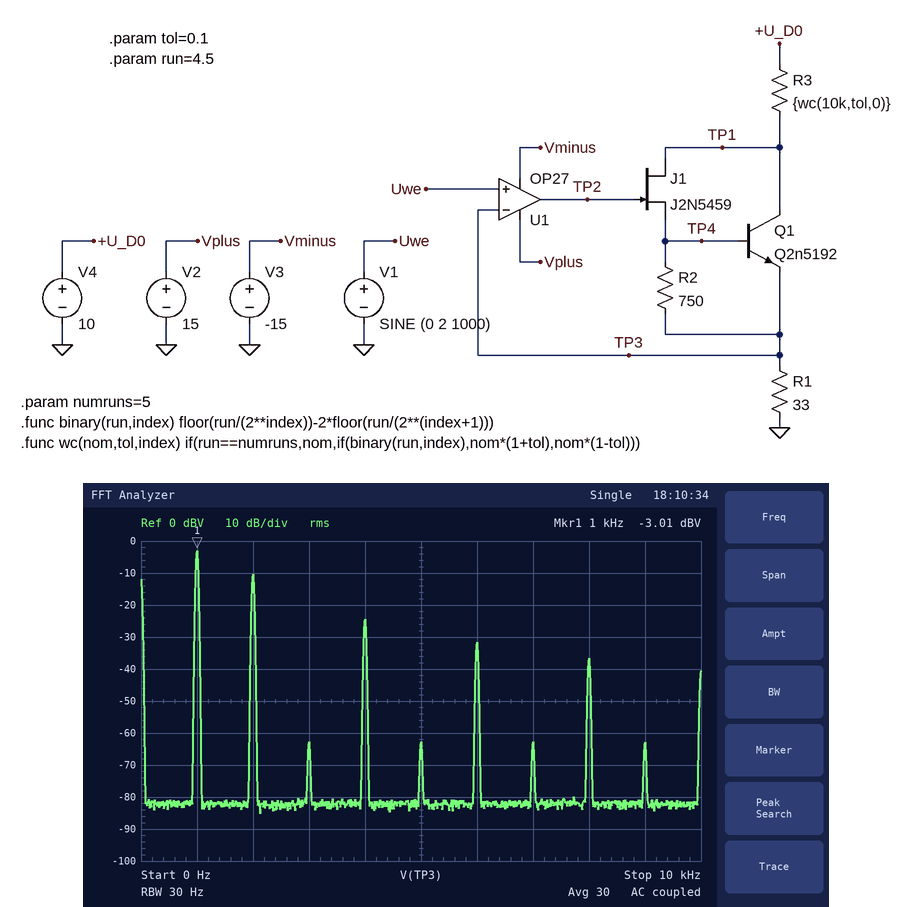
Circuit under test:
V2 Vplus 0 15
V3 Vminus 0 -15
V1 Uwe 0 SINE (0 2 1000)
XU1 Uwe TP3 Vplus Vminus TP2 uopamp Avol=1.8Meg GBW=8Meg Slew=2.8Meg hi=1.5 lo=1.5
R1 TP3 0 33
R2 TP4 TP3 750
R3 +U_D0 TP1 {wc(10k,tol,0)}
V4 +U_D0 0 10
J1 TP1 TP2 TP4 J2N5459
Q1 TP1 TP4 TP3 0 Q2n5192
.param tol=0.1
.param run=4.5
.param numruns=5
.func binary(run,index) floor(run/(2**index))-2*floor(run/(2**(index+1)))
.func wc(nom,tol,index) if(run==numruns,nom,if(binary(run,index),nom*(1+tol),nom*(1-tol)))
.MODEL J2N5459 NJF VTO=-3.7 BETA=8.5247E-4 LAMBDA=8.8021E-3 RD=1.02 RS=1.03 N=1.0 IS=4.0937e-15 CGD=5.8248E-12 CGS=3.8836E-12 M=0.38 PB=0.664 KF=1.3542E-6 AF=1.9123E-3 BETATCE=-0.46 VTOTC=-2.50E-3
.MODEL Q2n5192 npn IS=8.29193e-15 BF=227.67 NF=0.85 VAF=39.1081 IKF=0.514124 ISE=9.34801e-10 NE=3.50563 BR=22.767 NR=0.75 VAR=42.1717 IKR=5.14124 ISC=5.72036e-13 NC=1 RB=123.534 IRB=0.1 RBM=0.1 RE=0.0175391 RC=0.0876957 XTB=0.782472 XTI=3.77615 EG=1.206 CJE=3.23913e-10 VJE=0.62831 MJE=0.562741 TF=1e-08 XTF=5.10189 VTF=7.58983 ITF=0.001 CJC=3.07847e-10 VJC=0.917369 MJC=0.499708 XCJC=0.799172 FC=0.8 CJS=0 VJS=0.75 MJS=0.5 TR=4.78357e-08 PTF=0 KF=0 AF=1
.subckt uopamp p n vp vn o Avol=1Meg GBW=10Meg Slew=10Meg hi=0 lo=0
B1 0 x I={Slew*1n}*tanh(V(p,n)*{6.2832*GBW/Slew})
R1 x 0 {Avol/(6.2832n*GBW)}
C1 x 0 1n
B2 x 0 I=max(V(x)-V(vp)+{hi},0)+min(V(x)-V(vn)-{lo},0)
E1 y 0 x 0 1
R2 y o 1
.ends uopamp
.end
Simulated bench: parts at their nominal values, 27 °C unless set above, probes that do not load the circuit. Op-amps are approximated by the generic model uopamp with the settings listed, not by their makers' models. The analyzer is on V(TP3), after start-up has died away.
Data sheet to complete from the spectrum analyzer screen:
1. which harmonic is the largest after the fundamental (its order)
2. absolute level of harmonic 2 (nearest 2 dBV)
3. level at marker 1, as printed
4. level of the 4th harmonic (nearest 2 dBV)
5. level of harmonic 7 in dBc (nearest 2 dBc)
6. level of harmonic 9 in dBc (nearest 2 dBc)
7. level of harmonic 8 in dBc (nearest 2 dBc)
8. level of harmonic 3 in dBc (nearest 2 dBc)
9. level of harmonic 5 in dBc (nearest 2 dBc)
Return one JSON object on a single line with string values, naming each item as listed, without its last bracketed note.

{"which harmonic is the largest after the fundamental": "2", "absolute level of harmonic 2": "-10 dBV", "level at marker 1, as printed": "-3.01 dBV", "level of the 4th harmonic": "-24 dBV", "level of harmonic 7 in dBc": "-60 dBc", "level of harmonic 9 in dBc": "-60 dBc", "level of harmonic 8 in dBc": "-34 dBc", "level of harmonic 3 in dBc": "-60 dBc", "level of harmonic 5 in dBc": "-60 dBc"}
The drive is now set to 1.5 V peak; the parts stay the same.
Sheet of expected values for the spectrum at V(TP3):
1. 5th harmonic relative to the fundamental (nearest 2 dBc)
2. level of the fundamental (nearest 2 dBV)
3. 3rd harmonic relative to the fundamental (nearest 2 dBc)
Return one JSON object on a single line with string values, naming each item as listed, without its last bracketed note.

{"5th harmonic relative to the fundamental": "-58 dBc", "level of the fundamental": "-6 dBV", "3rd harmonic relative to the fundamental": "-58 dBc"}
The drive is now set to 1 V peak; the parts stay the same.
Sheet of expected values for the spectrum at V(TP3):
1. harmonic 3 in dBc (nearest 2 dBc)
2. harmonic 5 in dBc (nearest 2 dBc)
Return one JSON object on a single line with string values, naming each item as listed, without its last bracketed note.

{"harmonic 3 in dBc": "-54 dBc", "harmonic 5 in dBc": "-54 dBc"}
